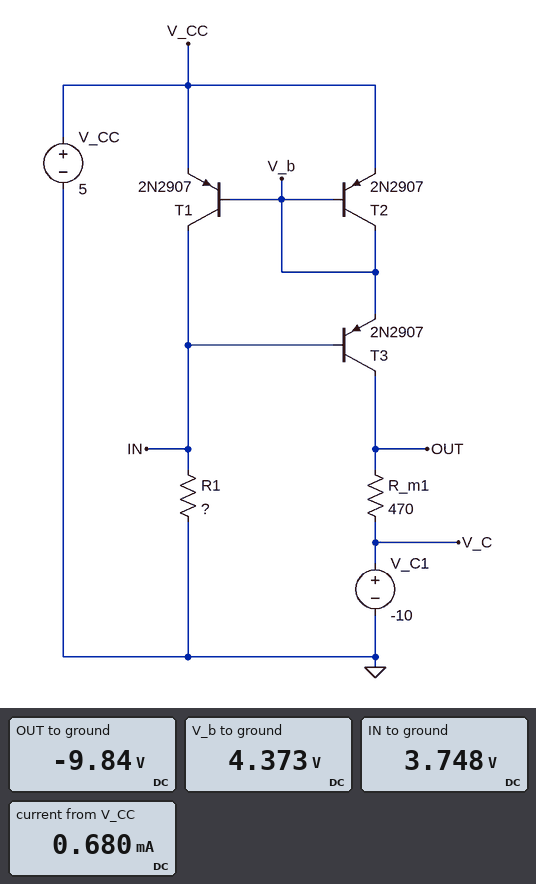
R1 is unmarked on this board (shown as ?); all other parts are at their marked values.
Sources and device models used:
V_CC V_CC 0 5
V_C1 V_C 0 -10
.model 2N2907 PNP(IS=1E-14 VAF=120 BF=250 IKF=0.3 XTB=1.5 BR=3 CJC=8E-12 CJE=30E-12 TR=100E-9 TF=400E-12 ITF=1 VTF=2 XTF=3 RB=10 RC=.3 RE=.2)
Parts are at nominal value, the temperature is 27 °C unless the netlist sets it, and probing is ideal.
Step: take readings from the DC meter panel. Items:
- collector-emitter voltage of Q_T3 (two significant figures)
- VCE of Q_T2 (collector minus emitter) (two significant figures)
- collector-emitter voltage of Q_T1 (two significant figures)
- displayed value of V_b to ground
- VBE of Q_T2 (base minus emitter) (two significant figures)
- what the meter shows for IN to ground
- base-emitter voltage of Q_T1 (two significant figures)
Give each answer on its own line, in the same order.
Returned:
-14 V
-630 mV
-1.3 V
4.373 V
-630 mV
3.748 V
-630 mV
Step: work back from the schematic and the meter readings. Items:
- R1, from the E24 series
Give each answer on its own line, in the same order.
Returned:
11 kΩ
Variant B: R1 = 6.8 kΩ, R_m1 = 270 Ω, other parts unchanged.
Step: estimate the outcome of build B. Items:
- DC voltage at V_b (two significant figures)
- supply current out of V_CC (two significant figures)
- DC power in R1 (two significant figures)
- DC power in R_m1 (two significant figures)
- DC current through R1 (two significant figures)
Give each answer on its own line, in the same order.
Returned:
4.4 V
1.1 mA
2.0 mW
80 µW
550 µA
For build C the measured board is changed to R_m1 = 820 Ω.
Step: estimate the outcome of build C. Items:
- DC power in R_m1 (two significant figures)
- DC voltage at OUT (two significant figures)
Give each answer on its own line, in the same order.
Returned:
94 µW
-9.7 V
